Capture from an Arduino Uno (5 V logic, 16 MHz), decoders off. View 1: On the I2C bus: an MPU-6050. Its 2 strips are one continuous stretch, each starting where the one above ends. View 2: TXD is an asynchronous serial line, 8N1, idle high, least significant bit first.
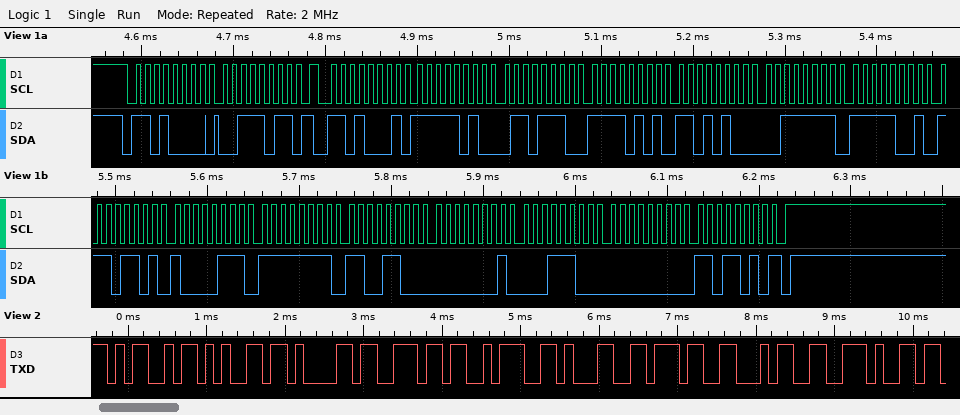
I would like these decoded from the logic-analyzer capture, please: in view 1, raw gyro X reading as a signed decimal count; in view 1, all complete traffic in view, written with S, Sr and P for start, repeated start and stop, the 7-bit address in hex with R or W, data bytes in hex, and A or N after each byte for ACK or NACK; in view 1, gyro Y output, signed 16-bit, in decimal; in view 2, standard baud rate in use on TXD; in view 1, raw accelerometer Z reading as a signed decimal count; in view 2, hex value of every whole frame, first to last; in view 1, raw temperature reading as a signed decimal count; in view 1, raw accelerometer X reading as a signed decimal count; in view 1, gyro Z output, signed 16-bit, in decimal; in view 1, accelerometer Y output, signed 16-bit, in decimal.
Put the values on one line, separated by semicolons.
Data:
-52; S 68W A 3B A Sr 68R A FA A 6E A F5 A D4 A 3F A F9 A ED A 87 A FF A CC A 01 A 1C A 00 A DA N P; 284; 9600 baud; 16377; 0x4D 0x65 0x61 0x6E 0x3A 0x31 0x37 0x34 0x2E; -4729; -1426; 218; -2604
